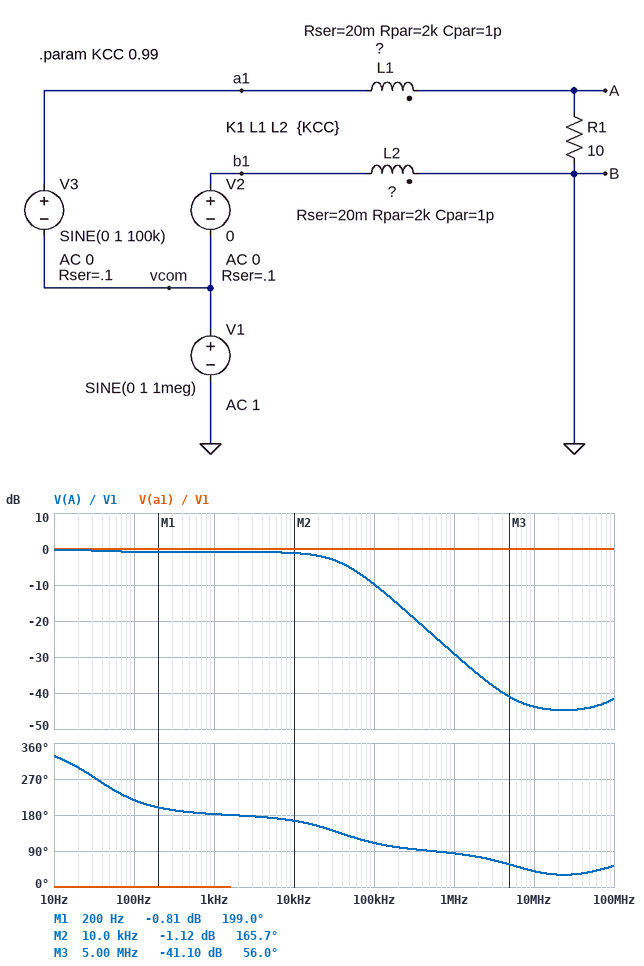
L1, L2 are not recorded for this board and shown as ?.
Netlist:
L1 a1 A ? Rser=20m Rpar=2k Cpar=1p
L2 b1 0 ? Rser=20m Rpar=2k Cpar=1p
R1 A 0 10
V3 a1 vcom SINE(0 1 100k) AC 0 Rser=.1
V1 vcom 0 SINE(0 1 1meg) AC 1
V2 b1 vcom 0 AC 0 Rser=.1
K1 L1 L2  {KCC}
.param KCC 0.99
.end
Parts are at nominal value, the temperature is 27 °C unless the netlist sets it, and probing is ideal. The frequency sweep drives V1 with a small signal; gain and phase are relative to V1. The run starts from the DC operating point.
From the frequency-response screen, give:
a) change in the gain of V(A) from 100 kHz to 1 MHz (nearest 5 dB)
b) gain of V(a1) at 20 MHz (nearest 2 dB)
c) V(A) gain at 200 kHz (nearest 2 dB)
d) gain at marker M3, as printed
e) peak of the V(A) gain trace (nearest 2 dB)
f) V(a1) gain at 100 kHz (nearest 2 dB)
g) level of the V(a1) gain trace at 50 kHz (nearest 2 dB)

-20 dB
0 dB
-16 dB
-41.10 dB
0 dB
0 dB
0 dB
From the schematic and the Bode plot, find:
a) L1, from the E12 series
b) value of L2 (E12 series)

2.2 mH
560 µH
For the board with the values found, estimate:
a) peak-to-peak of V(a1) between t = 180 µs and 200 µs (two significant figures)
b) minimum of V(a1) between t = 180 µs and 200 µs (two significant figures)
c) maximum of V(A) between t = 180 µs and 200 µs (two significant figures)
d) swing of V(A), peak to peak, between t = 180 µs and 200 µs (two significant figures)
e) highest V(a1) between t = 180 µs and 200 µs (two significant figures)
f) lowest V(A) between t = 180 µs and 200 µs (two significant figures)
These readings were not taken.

4.0 V
-2.0 V
360 mV
740 mV
2.0 V
-370 mV
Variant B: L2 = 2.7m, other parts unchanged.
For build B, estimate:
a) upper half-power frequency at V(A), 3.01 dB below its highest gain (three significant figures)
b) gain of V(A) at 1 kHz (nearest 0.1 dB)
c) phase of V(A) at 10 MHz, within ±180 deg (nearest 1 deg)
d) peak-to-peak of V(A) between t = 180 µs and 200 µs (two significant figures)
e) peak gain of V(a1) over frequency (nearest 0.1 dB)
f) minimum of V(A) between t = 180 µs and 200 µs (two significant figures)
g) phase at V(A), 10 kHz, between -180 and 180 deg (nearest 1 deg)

7.09 Hz
-19.6 dB
3 deg
680 mV
0 dB
-340 mV
-15 deg
